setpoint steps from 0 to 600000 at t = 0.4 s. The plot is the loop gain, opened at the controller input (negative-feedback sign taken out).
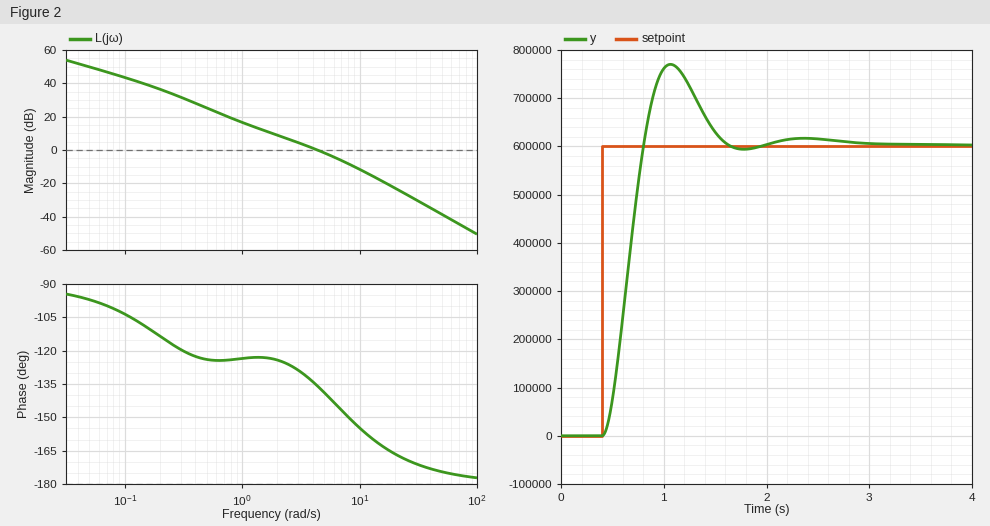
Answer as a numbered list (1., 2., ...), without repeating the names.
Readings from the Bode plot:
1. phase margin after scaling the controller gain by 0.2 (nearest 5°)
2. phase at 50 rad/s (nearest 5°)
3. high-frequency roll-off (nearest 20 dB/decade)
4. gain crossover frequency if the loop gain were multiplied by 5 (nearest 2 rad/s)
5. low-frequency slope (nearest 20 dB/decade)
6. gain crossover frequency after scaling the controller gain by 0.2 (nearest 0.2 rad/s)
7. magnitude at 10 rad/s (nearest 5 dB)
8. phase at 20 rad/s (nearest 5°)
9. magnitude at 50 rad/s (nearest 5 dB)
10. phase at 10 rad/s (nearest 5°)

1. 55°
2. -175°
3. -40 dB/decade
4. 12 rad/s
5. -20 dB/decade
6. 1.2 rad/s
7. -10 dB
8. -165°
9. -40 dB
10. -155°
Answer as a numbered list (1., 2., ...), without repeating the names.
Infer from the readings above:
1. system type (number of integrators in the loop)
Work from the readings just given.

1. 1
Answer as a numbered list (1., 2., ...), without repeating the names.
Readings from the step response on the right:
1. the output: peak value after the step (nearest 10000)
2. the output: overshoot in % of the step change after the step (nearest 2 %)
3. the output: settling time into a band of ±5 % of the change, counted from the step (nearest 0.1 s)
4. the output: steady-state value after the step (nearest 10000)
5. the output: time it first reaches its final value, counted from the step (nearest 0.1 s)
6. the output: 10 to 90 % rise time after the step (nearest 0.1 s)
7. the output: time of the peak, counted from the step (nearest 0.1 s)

1. 770000
2. 28 %
3. 1.1 s
4. 600000
5. 0.4 s
6. 0.3 s
7. 0.7 s
